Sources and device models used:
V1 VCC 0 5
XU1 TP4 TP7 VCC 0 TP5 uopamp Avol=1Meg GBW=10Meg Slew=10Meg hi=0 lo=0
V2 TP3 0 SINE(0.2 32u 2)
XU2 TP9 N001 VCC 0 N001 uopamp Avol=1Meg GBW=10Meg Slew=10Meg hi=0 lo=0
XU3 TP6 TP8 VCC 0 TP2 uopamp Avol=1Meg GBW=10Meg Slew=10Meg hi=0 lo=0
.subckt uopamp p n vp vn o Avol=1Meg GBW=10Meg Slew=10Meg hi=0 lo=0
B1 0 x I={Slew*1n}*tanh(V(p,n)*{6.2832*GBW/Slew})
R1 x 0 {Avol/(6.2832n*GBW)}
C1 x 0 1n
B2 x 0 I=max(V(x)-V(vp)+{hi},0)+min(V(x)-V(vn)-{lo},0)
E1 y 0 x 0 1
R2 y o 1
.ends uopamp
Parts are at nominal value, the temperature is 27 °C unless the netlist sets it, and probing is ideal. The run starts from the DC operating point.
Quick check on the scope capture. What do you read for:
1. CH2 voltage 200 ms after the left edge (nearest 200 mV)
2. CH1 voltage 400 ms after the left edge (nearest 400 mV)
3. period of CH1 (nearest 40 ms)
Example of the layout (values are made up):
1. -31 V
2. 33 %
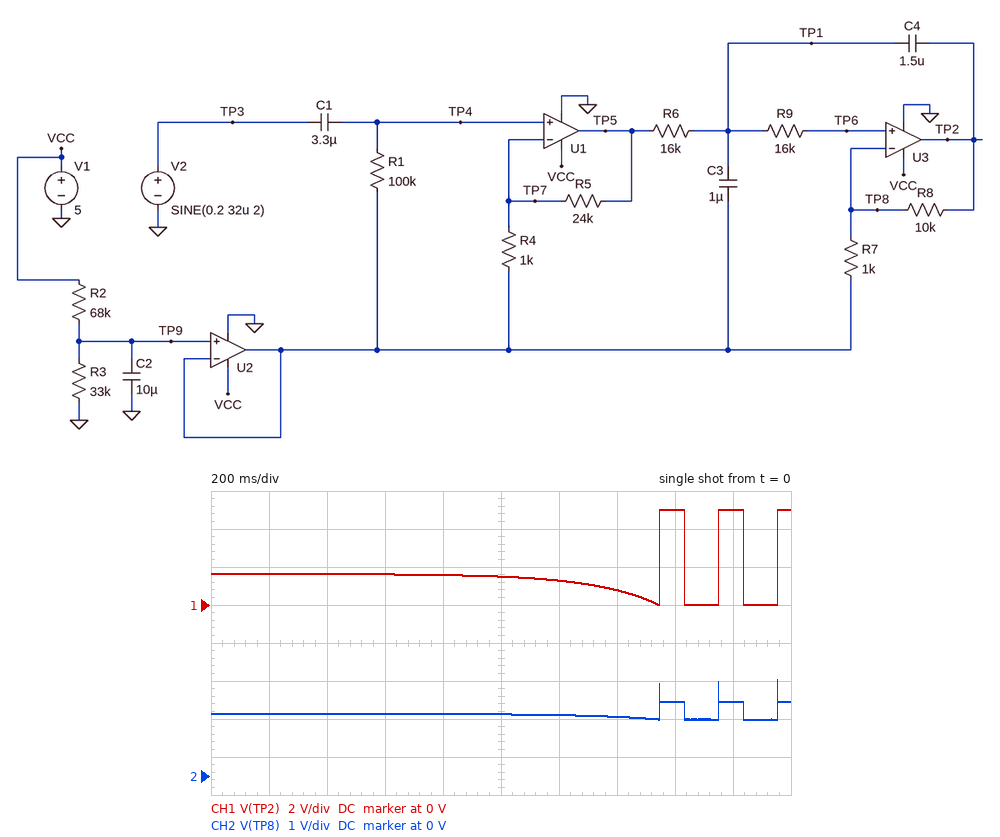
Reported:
1. 1.6 V
2. 1.6 V
3. 200 ms
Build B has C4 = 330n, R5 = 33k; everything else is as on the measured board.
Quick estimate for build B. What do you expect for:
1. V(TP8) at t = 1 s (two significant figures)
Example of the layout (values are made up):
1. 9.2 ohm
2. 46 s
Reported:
1. 1.5 V
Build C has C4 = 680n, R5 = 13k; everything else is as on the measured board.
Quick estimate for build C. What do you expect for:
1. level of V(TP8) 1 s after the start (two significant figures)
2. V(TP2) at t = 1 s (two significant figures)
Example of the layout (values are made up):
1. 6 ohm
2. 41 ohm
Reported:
1. 1.9 V
2. 5.0 V
